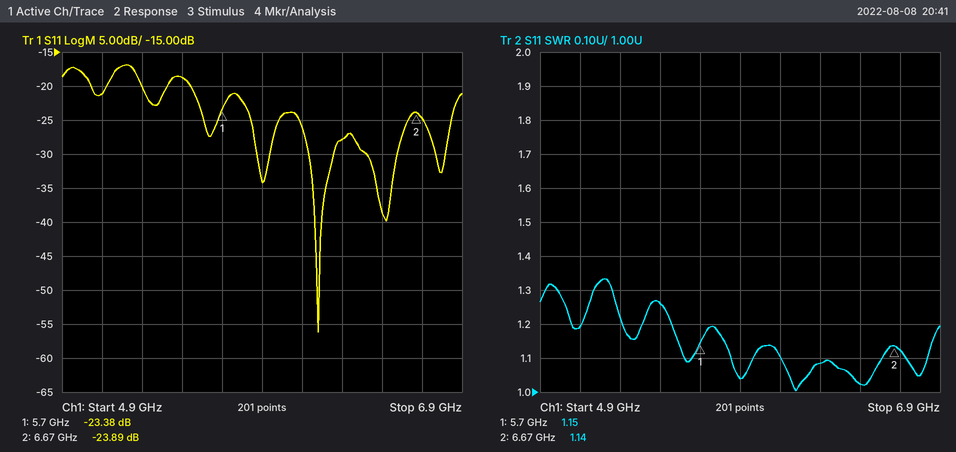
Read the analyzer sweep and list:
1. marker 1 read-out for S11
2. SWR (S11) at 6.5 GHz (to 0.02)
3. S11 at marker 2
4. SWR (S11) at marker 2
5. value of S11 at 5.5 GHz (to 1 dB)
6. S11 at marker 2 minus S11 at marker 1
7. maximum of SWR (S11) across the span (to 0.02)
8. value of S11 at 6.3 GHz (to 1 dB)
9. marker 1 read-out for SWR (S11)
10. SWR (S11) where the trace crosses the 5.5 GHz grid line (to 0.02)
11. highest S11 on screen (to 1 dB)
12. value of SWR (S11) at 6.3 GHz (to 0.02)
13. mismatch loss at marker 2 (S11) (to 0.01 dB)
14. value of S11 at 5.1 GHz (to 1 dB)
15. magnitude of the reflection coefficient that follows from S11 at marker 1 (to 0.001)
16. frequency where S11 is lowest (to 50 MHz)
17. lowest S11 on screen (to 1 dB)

-23.38 dB
1.02
-23.89 dB
1.14
-19 dB
-0.51 dB
1.34
-28 dB
1.15
1.26
-17 dB
1.08
0.02 dB
-21 dB
0.068
6.20 GHz
-56 dB
